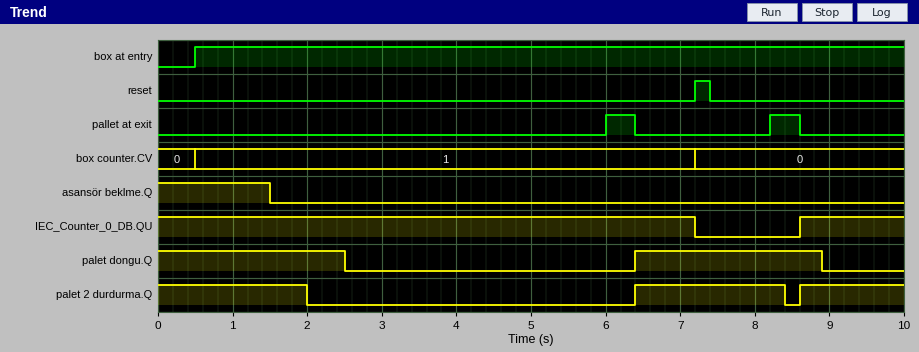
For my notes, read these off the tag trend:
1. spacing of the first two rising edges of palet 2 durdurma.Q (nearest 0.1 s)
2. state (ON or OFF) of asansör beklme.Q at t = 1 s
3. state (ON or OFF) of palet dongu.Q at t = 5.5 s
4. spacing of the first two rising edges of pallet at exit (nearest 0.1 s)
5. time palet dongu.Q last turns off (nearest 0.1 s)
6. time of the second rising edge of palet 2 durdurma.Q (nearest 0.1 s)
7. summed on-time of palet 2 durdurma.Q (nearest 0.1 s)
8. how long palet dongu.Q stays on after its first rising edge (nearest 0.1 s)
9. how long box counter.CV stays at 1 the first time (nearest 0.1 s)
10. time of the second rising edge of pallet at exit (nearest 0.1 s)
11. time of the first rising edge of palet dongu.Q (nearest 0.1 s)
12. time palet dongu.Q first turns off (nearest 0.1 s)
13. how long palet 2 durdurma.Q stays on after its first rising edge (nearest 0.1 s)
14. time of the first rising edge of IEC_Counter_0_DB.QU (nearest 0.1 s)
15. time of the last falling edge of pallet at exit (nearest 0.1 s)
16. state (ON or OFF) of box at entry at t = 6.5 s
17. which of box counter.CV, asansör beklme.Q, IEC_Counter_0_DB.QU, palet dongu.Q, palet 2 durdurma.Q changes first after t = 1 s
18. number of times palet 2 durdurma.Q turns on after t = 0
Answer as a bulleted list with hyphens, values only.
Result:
- 2.2 s
- ON
- OFF
- 2.2 s
- 8.9 s
- 8.6 s
- 5.4 s
- 2.5 s
- 6.7 s
- 8.2 s
- 6.4 s
- 2.5 s
- 2.0 s
- 8.6 s
- 8.6 s
- ON
- asansör beklme.Q
- 2
